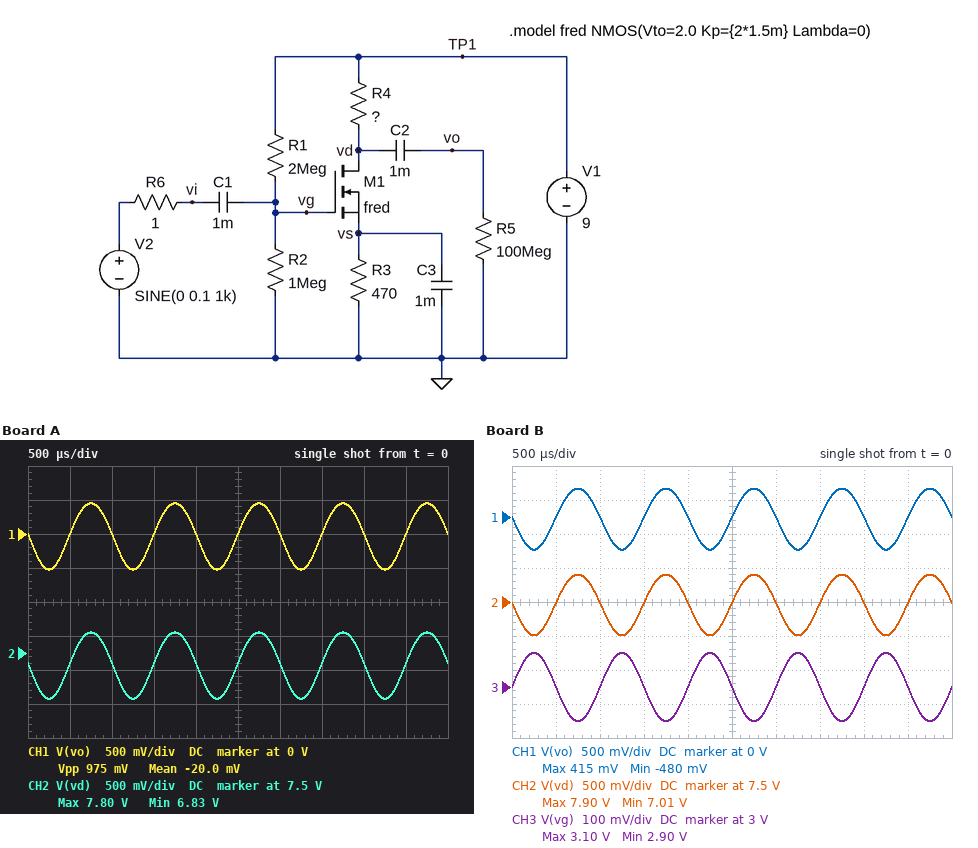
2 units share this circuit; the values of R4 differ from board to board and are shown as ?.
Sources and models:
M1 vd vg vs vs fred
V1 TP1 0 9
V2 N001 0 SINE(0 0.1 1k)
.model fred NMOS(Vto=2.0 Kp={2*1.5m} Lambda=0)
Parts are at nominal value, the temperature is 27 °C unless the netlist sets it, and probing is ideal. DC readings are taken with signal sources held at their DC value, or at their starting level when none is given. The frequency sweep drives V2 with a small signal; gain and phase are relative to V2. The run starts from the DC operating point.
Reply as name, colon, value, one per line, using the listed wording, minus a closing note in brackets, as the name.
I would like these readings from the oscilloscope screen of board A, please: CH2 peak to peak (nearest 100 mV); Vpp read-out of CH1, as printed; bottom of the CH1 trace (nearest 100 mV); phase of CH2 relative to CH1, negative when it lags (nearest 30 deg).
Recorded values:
CH2 peak to peak: 1.0 V
Vpp read-out of CH1, as printed: 975 mV
bottom of the CH1 trace: -500 mV
phase of CH2 relative to CH1, negative when it lags: 0 deg
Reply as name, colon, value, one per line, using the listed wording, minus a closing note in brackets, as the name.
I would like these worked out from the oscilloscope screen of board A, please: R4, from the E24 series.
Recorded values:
R4, from the E24 series: 2.4 kΩ
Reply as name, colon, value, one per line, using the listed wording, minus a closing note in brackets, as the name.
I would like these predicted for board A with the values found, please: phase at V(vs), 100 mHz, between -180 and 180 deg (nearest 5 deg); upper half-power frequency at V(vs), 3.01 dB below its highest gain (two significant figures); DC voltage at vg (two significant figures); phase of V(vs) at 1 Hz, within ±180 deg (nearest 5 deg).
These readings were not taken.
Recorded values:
phase at V(vs), 100 mHz, between -180 and 180 deg: -10 deg
upper half-power frequency at V(vs), 3.01 dB below its highest gain: 660 mHz
DC voltage at vg: 3.0 V
phase of V(vs) at 1 Hz, within ±180 deg: -55 deg
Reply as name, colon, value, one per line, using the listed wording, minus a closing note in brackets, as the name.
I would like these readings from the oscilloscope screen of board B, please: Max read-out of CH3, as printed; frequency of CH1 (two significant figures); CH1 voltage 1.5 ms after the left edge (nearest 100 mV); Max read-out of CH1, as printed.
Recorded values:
Max read-out of CH3, as printed: 3.10 V
frequency of CH1: 1.0 kHz
CH1 voltage 1.5 ms after the left edge: 0 V
Max read-out of CH1, as printed: 415 mV
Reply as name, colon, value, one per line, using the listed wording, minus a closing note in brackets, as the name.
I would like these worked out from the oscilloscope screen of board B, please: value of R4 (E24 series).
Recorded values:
value of R4: 2.2 kΩ
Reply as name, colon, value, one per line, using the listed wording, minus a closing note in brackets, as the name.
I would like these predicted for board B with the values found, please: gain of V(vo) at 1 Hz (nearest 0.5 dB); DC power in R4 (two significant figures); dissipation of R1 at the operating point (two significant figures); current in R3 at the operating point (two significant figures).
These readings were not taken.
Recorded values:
gain of V(vo) at 1 Hz: 12.0 dB
DC power in R4: 1.0 mW
dissipation of R1 at the operating point: 18 µW
current in R3 at the operating point: 690 µA
